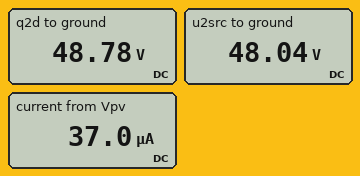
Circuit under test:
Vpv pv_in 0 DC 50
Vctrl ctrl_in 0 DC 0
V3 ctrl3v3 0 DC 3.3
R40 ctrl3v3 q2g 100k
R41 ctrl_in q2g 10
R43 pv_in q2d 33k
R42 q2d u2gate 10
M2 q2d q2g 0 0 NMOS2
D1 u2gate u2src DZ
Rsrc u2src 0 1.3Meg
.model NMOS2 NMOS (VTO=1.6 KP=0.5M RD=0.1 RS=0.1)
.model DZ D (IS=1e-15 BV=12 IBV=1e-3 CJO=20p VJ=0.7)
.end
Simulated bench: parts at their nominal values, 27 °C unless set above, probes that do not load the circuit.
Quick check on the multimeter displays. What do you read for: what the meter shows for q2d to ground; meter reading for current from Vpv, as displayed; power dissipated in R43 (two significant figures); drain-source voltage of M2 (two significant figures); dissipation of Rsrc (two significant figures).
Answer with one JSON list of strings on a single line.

["48.78 V", "37.0 µA", "45 µW", "49 V", "1.8 mW"]
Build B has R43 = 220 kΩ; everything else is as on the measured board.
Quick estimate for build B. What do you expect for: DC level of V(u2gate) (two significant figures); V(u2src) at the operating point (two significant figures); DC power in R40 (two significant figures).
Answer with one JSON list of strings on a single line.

["43 V", "42 V", "110 µW"]
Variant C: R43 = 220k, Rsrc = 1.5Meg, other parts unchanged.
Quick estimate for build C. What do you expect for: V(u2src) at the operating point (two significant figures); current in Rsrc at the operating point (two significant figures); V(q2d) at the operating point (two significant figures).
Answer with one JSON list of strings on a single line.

["43 V", "29 µA", "44 V"]
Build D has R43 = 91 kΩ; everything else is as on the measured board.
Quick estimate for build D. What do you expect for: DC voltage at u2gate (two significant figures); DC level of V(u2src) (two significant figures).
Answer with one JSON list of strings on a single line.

["47 V", "46 V"]
